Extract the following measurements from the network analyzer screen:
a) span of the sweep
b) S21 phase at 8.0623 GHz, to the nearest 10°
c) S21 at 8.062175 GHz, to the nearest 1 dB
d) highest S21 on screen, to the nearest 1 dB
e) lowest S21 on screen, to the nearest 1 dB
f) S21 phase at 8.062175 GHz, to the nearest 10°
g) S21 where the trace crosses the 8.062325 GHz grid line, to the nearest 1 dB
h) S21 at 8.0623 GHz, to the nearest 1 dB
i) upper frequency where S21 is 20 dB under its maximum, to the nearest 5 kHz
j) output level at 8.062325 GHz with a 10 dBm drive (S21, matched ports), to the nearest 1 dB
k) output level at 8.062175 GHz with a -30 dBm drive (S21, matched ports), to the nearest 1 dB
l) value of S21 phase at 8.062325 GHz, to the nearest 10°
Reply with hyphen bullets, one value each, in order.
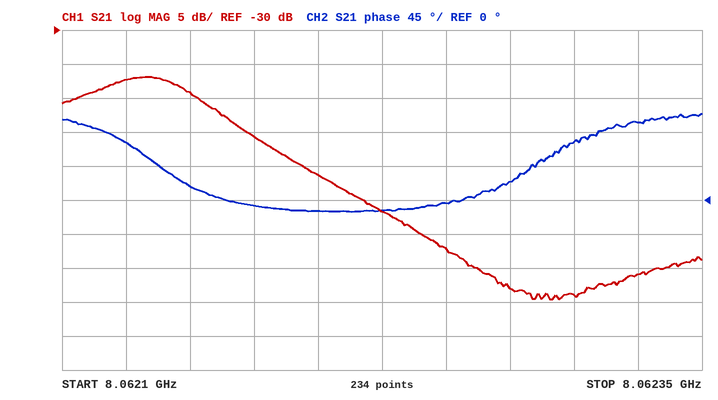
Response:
- 250 kHz
- 80°
- -46 dB
- -37 dB
- -70 dB
- -10°
- -66 dB
- -69 dB
- 8.062225 GHz
- -56 dBm
- -76 dBm
- 100°
